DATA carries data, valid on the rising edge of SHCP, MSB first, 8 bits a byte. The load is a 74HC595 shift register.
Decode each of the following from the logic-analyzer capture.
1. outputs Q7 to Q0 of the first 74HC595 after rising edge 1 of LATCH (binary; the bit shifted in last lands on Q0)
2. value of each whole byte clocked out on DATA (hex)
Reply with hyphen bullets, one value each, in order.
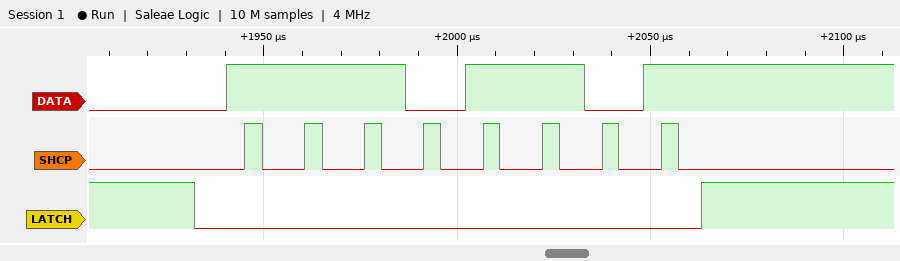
- 11101101
- ED
